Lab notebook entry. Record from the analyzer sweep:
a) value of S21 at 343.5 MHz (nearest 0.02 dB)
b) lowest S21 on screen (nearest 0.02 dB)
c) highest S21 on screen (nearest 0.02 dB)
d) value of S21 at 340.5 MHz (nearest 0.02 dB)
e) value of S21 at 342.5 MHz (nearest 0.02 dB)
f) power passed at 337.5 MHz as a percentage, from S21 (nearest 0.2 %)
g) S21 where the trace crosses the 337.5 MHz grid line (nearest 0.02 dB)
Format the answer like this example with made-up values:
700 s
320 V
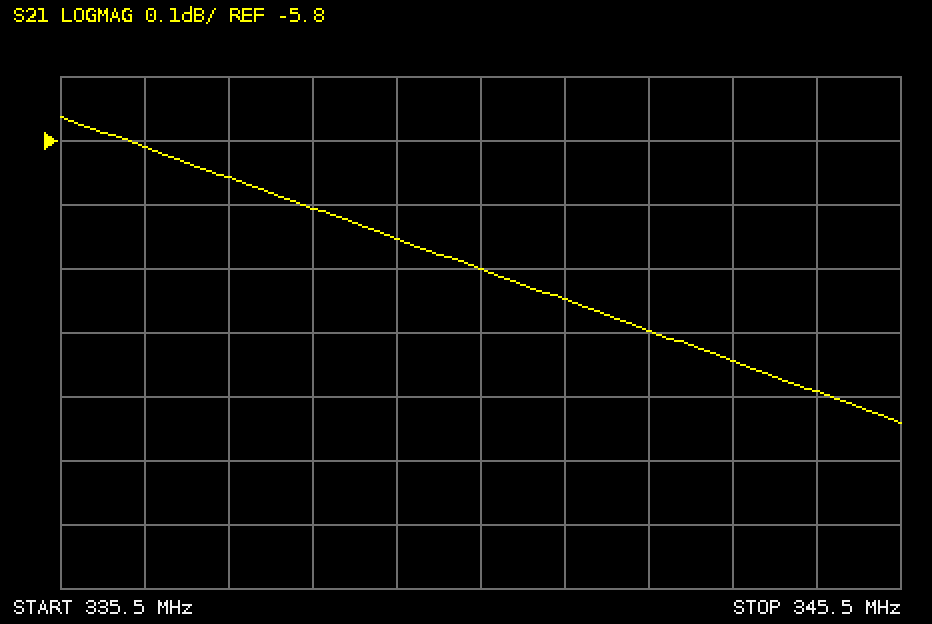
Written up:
-6.14 dB
-6.24 dB
-5.76 dB
-6.00 dB
-6.10 dB
26.0 %
-5.86 dB
